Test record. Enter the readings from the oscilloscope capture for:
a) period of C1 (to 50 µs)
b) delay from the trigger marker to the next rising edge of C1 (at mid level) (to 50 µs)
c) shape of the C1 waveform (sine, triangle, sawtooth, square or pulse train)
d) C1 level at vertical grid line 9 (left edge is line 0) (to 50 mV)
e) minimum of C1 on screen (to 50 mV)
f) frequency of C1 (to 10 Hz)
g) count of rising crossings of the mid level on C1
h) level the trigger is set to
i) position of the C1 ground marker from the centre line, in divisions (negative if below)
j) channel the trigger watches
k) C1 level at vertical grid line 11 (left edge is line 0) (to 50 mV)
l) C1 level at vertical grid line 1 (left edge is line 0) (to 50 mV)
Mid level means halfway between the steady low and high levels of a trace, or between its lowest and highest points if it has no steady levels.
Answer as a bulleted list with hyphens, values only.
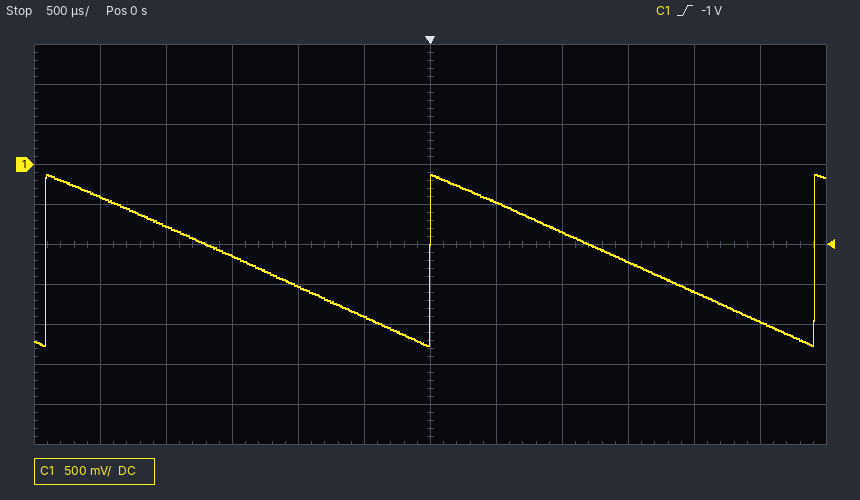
- 2.90 ms
- 2.90 ms
- sawtooth
- -1.20 V
- -2.25 V
- 340 Hz
- 3
- -1 V
- +2.0 div
- C1
- -1.95 V
- -400 mV
